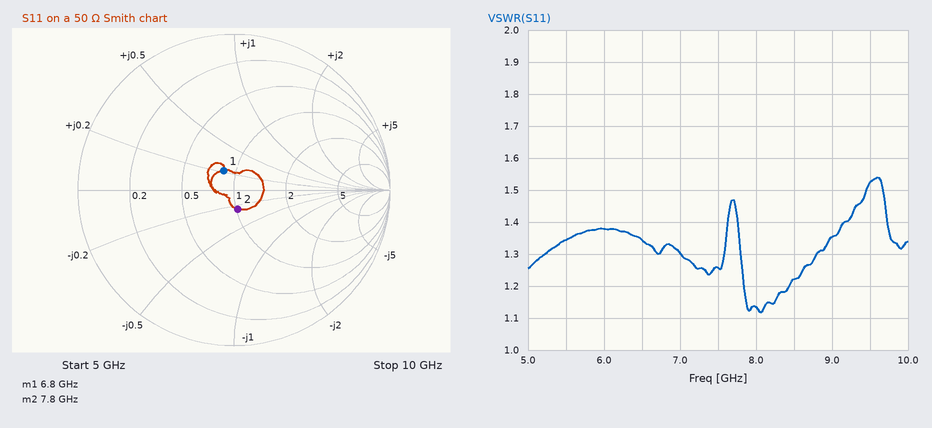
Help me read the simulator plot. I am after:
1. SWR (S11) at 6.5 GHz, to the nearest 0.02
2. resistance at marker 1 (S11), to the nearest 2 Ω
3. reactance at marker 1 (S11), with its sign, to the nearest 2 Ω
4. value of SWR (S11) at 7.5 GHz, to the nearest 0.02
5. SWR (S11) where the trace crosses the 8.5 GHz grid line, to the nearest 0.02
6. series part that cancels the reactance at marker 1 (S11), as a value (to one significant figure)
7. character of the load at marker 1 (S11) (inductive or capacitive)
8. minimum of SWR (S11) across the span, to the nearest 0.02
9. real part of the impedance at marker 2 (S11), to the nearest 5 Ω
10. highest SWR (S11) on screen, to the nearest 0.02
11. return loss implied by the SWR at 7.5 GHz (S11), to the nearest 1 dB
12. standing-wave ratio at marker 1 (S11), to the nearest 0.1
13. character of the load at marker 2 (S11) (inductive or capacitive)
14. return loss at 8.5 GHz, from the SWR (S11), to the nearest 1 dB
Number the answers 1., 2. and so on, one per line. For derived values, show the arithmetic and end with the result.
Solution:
1. 1.34
2. 42 Ω
3. +10 Ω
4. 1.26
5. 1.22
6. C = 1/(2π × 6.8 GHz × 10 Ω) ≈ 2 pF
7. inductive
8. 1.12
9. 50 Ω
10. 1.54
11. −20 log10((1.26 − 1)/(1.26 + 1)) ≈ 19 dB
12. 1.3
13. capacitive
14. −20 log10((1.22 − 1)/(1.22 + 1)) ≈ 20 dB
